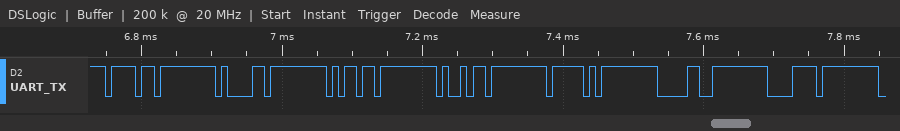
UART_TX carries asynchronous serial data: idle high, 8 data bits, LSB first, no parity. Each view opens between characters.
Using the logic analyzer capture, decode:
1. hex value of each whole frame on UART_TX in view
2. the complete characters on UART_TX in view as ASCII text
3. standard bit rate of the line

6F, 61, 6D, 69, 5F, 30, 78
"oami_0x"
115200 baud
